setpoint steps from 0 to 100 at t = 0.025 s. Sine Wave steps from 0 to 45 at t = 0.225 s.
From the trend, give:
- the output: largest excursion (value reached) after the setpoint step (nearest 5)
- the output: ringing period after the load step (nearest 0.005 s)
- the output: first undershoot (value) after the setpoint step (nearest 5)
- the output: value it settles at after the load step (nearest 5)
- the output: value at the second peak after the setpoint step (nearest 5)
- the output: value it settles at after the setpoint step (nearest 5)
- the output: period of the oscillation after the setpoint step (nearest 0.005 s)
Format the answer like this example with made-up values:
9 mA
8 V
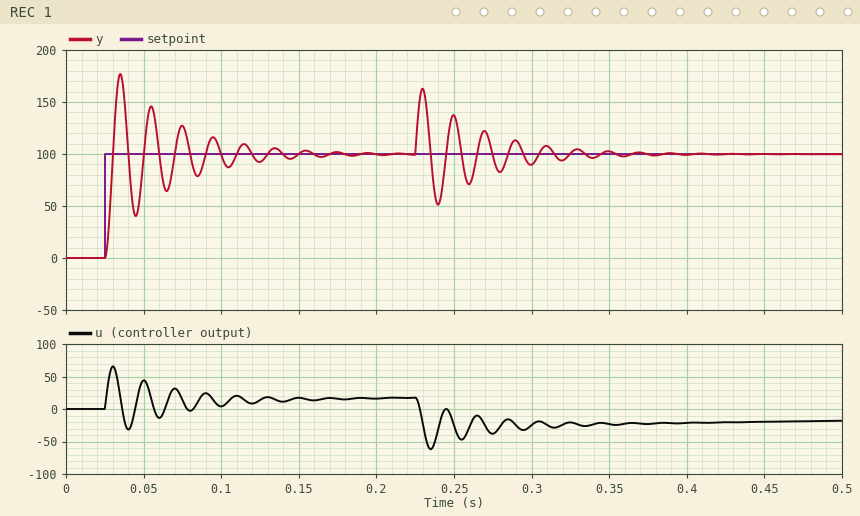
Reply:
175
0.020 s
40
100
145
100
0.020 s
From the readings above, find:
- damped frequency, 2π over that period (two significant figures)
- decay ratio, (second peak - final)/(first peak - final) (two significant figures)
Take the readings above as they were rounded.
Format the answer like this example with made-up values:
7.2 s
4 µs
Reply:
310 rad/s
0.60
